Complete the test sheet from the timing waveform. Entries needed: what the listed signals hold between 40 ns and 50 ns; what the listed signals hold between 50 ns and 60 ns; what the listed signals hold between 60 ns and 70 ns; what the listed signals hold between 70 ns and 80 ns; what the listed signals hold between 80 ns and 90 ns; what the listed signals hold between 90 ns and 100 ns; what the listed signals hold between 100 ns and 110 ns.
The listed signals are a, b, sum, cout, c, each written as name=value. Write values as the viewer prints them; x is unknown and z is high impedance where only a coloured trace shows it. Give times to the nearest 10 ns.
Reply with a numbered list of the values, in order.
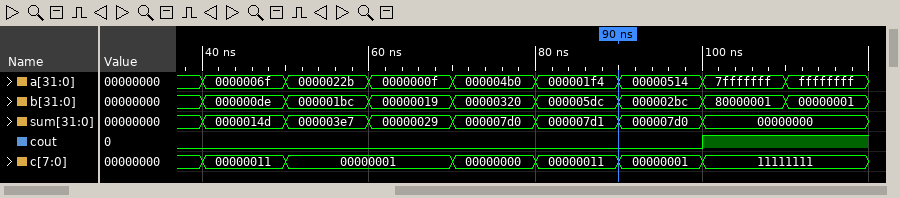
1. a=0000006f, b=000000de, sum=0000014d, cout=0, c=00000011
2. a=0000022b, b=000001bc, sum=000003e7, cout=0, c=00000001
3. a=0000000f, b=00000019, sum=00000029, cout=0, c=00000001
4. a=000004b0, b=00000320, sum=000007d0, cout=0, c=00000000
5. a=000001f4, b=000005dc, sum=000007d1, cout=0, c=00000011
6. a=00000514, b=000002bc, sum=000007d0, cout=0, c=00000001
7. a=7fffffff, b=80000001, sum=00000000, cout=1, c=11111111
